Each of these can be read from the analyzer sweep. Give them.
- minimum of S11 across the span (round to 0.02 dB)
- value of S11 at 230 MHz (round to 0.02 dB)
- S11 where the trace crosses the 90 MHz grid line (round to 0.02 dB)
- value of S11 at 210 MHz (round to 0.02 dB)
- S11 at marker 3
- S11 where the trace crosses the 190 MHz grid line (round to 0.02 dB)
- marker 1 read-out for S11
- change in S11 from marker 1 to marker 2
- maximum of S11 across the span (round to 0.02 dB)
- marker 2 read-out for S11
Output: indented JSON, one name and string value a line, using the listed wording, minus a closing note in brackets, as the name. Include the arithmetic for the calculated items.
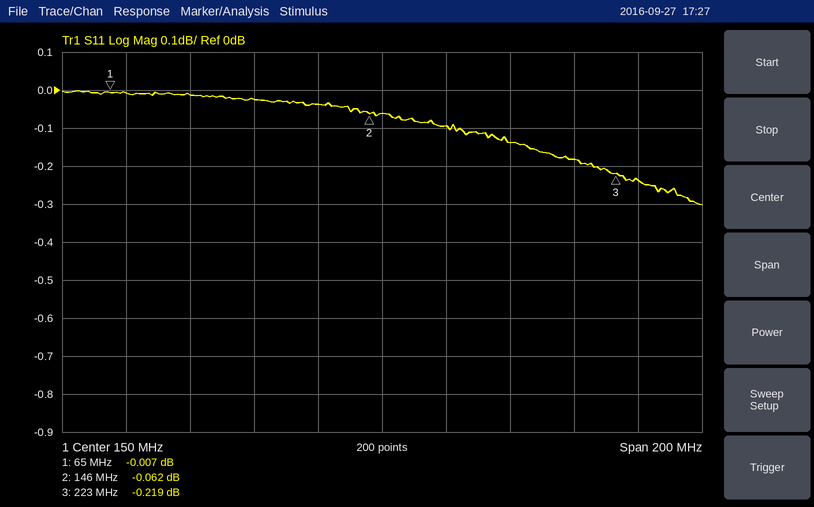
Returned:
{
  "minimum of S11 across the span": "-0.30 dB",
  "value of S11 at 230 MHz": "-0.24 dB",
  "S11 where the trace crosses the 90 MHz grid line": "-0.02 dB",
  "value of S11 at 210 MHz": "-0.18 dB",
  "S11 at marker 3": "-0.219 dB",
  "S11 where the trace crosses the 190 MHz grid line": "-0.14 dB",
  "marker 1 read-out for S11": "-0.007 dB",
  "change in S11 from marker 1 to marker 2": "-0.062 − (-0.007) = -0.055 dB",
  "maximum of S11 across the span": "0.00 dB",
  "marker 2 read-out for S11": "-0.062 dB"
}
